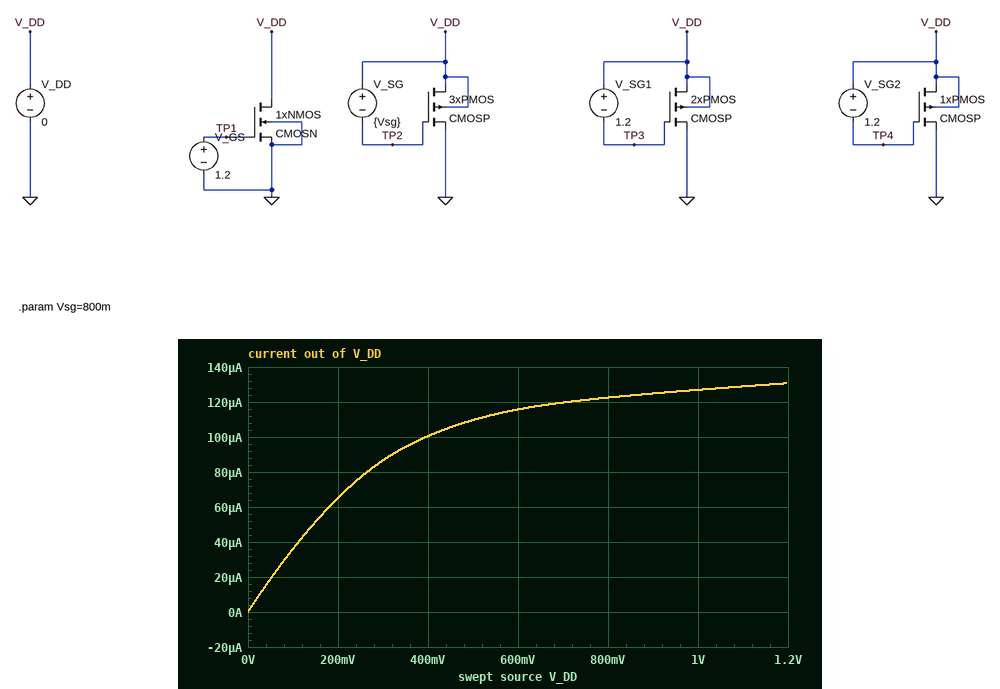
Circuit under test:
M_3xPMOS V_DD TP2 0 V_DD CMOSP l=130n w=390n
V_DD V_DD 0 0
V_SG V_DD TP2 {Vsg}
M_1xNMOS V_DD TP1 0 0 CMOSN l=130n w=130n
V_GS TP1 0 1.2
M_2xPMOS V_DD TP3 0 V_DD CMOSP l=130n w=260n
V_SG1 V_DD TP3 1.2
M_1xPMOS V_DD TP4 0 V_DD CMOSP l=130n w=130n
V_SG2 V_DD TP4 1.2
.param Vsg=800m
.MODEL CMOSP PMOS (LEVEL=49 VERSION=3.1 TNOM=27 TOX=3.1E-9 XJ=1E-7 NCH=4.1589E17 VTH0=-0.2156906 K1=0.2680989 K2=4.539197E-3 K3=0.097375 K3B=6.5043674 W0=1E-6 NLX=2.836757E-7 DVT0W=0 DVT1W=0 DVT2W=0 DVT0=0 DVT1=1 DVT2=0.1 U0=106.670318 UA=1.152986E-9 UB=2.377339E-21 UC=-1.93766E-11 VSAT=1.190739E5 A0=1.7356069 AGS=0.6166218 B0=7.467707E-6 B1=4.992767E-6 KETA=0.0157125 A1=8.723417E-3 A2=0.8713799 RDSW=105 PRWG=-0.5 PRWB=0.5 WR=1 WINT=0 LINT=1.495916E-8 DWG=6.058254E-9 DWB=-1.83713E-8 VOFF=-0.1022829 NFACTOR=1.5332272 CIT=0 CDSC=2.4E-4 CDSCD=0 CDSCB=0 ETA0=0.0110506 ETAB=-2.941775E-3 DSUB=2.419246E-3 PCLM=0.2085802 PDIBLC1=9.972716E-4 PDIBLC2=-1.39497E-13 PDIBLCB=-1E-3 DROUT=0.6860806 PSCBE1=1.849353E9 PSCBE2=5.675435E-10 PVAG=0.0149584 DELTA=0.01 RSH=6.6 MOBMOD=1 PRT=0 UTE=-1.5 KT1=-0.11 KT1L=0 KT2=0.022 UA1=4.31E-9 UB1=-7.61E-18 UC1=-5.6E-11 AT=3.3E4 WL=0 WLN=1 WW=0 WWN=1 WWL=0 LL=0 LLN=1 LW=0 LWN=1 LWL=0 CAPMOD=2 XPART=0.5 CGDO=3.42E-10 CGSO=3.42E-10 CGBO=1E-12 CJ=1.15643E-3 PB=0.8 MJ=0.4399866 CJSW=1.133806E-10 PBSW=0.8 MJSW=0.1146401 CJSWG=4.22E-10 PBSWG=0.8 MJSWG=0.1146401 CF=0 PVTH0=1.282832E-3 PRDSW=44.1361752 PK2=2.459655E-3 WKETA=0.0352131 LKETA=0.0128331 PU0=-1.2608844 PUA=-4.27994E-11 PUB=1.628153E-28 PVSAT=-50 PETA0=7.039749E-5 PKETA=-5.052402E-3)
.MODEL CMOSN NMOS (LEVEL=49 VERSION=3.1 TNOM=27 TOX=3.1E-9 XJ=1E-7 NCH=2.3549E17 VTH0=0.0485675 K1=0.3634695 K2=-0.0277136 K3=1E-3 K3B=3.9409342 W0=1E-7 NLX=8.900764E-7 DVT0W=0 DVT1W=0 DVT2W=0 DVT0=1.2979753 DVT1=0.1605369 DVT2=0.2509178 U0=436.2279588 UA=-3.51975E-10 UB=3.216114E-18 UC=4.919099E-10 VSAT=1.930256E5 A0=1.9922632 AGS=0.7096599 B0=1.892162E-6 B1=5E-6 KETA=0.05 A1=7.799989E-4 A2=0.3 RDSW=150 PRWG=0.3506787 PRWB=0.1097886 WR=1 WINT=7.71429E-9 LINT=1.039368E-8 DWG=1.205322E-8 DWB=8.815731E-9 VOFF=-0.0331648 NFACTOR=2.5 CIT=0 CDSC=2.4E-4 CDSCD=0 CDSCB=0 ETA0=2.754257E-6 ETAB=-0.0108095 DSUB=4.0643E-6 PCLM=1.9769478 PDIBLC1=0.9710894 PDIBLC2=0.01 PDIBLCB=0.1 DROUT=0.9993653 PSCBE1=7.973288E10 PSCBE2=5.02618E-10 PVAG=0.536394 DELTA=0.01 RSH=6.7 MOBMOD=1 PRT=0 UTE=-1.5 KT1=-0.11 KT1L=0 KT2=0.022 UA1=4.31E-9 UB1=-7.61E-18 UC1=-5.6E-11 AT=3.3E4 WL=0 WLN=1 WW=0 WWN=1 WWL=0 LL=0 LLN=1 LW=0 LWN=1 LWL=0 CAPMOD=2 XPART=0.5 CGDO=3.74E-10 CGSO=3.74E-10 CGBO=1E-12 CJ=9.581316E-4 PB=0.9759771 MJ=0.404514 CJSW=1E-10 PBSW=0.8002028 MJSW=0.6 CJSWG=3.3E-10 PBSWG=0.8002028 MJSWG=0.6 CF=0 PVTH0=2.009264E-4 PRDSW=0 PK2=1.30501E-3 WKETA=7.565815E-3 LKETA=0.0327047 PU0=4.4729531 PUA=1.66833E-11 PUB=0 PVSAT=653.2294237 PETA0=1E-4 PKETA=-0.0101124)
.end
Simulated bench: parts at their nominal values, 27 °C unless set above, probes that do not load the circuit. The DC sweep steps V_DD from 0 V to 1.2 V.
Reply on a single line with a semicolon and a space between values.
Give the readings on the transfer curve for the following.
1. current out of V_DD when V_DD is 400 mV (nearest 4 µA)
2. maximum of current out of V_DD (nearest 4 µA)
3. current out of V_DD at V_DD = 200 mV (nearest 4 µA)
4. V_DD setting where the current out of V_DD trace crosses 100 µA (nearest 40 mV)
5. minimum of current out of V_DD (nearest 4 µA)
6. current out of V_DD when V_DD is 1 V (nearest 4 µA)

100 µA; 132 µA; 64 µA; 400 mV; 0 A; 128 µA
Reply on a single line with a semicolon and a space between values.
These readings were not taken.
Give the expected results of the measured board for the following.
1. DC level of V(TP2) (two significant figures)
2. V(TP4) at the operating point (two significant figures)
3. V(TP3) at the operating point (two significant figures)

-800 mV; -1.2 V; -1.2 V
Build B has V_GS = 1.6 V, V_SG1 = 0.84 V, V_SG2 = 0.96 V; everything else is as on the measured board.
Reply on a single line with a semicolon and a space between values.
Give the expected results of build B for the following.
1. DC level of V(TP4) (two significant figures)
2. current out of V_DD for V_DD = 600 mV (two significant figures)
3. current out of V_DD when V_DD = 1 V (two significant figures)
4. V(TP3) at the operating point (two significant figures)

-960 mV; 100 µA; 110 µA; -840 mV
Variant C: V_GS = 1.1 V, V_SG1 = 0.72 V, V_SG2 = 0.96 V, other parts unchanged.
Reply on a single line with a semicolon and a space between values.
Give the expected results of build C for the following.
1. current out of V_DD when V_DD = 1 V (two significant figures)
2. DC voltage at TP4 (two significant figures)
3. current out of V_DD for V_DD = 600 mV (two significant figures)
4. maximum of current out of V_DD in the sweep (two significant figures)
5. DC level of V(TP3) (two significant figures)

85 µA; -960 mV; 77 µA; 88 µA; -720 mV
